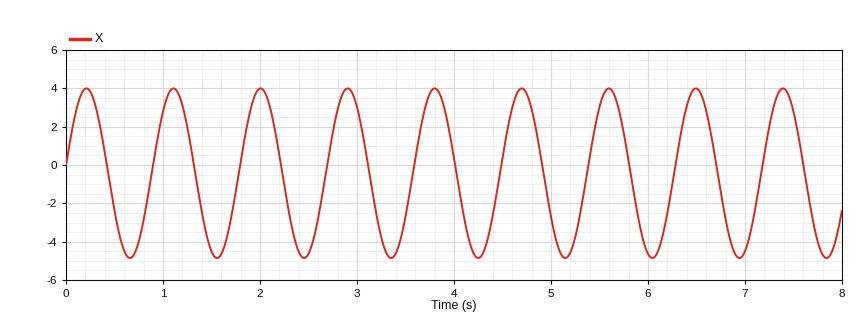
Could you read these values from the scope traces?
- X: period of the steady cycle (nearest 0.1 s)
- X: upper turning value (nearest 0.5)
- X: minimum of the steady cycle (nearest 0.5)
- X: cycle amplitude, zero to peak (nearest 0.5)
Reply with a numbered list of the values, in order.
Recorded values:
1. 0.9 s
2. 4.0
3. -5.0
4. 4.5
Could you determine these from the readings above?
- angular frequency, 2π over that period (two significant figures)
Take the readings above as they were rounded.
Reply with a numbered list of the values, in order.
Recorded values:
1. 7.0 rad/s
